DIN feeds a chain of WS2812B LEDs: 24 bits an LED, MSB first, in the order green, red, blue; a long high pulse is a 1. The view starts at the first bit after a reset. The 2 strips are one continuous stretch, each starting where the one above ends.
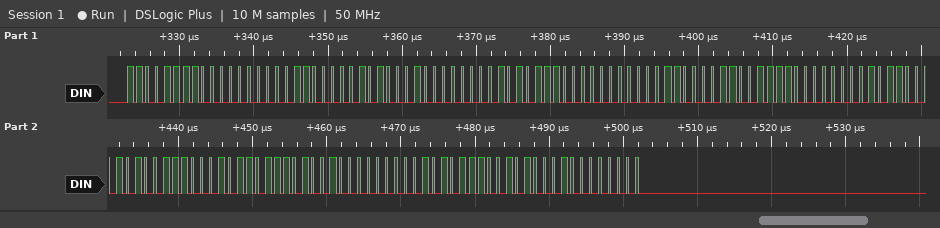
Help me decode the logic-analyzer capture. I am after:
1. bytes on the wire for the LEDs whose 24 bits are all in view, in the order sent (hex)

CF 00 30 51 00 AE 00 30 CF 00 B1 4E 2D D2 00 AE 51 00
